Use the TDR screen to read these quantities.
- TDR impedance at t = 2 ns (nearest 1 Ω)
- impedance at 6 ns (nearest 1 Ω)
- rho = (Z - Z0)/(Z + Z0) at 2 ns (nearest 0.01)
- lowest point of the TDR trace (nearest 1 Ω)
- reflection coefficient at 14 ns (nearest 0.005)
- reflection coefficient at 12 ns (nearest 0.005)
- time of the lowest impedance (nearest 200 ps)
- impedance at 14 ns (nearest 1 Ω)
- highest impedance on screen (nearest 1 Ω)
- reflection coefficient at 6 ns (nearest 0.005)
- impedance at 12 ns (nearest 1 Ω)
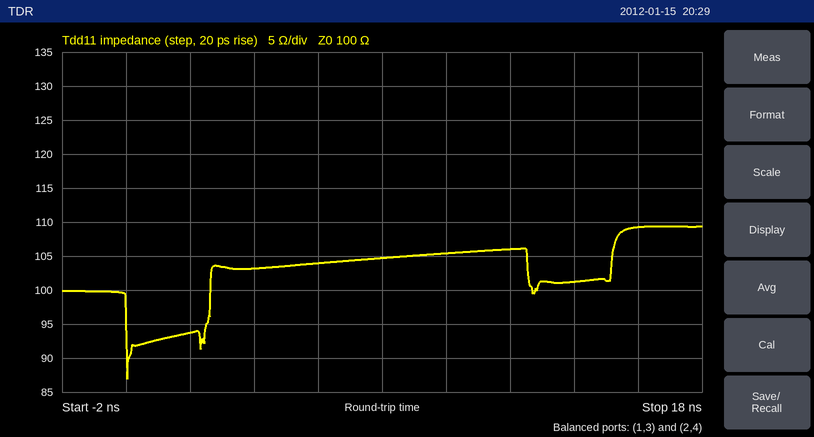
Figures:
94 Ω
104 Ω
-0.03
87 Ω
+0.005
+0.030
0.0 ns
101 Ω
109 Ω
+0.020
106 Ω
